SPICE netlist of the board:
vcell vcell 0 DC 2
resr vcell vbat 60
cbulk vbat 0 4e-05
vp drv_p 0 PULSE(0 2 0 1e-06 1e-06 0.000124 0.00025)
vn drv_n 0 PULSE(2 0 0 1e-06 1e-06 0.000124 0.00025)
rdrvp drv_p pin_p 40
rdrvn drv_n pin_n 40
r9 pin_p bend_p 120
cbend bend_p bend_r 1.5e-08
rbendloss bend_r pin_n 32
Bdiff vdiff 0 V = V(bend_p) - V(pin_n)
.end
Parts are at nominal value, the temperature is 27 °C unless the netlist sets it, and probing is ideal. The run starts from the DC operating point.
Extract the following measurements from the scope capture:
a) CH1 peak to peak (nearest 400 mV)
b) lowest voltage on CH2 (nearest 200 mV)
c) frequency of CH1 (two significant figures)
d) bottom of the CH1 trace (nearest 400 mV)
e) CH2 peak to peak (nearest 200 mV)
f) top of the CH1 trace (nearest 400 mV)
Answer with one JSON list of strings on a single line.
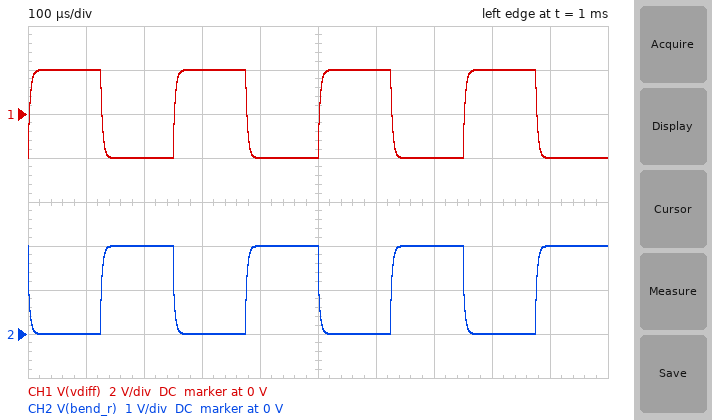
["4.0 V", "0 V", "4.0 kHz", "-2.0 V", "2.0 V", "2.0 V"]
